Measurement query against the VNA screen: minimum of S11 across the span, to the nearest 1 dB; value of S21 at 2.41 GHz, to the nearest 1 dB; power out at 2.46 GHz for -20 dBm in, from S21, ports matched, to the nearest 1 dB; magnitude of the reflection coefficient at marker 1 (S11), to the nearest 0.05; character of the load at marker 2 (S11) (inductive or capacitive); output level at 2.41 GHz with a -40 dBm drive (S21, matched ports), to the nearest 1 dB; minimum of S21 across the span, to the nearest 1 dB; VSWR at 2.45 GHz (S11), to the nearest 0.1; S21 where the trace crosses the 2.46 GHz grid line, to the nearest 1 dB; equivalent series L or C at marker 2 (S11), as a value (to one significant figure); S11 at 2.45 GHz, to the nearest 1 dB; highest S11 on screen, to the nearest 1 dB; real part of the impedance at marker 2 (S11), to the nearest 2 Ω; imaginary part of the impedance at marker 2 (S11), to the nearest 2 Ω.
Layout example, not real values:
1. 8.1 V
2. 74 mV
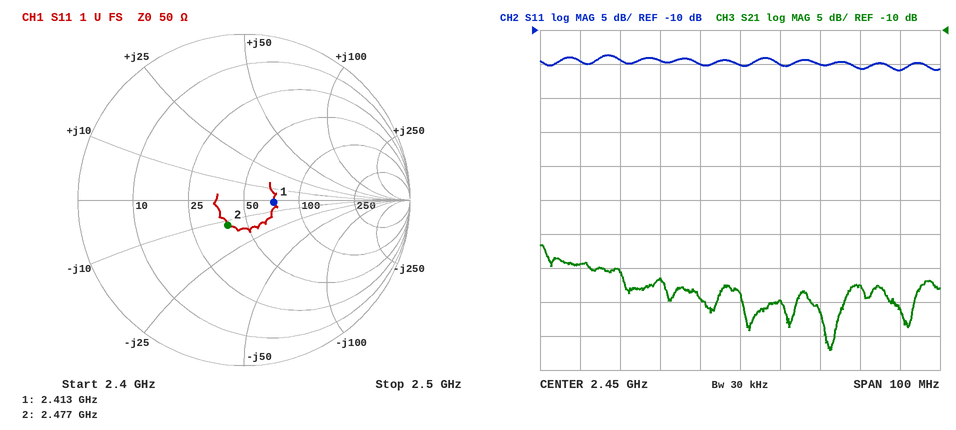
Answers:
1. -16 dB
2. -44 dB
3. -70 dBm
4. 0.20
5. capacitive
6. -84 dBm
7. -57 dB
8. 1.4
9. -50 dB
10. 5 pF
11. -15 dB
12. -14 dB
13. 40 Ω
14. -12 Ω
